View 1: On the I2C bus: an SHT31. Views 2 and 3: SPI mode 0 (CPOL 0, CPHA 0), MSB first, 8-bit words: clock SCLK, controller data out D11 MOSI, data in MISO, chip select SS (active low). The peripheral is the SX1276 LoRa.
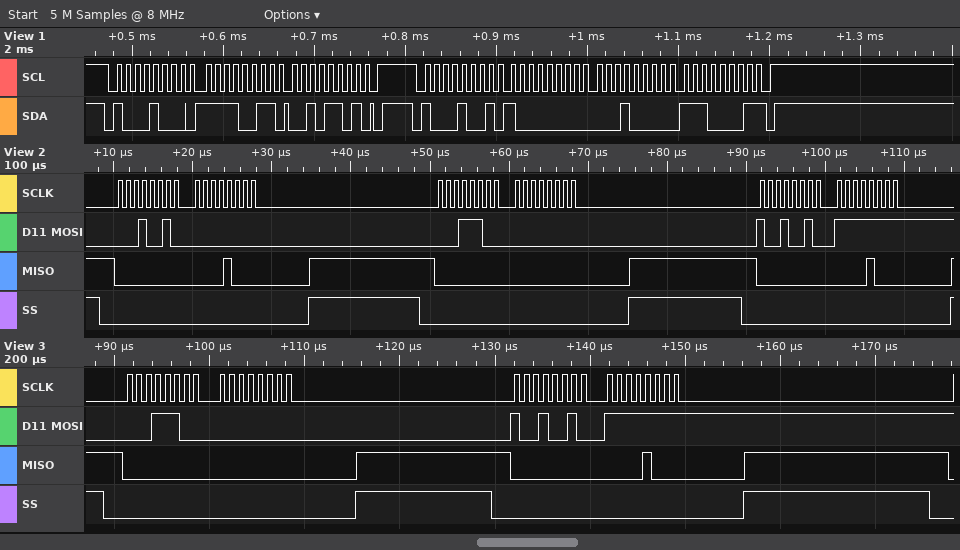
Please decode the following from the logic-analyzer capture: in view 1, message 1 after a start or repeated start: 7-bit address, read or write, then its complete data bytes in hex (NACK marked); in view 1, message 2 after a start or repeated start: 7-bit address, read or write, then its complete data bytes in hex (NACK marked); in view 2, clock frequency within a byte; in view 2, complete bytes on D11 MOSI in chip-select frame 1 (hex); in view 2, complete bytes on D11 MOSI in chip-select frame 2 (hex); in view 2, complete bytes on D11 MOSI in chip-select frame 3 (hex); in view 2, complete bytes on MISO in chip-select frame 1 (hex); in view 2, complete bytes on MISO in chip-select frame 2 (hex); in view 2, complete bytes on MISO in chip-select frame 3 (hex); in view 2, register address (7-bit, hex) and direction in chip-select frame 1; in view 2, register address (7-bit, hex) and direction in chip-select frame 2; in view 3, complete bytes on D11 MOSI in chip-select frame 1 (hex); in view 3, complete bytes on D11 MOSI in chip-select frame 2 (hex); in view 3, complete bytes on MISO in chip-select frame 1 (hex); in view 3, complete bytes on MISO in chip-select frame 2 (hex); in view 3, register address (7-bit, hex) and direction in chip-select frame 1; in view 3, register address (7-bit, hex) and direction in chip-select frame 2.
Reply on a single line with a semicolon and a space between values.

0x44 write: F3 2D; 0x44 read: 80 10 E1 NACK; 1 MHz; 12 00; 1C 00; 92 FF; 00 08; 00 00; 00 08; 0x12 read; 0x1C read; 1C 00; 92 FF; 00 00; 00 08; 0x1C read; 0x12 write
